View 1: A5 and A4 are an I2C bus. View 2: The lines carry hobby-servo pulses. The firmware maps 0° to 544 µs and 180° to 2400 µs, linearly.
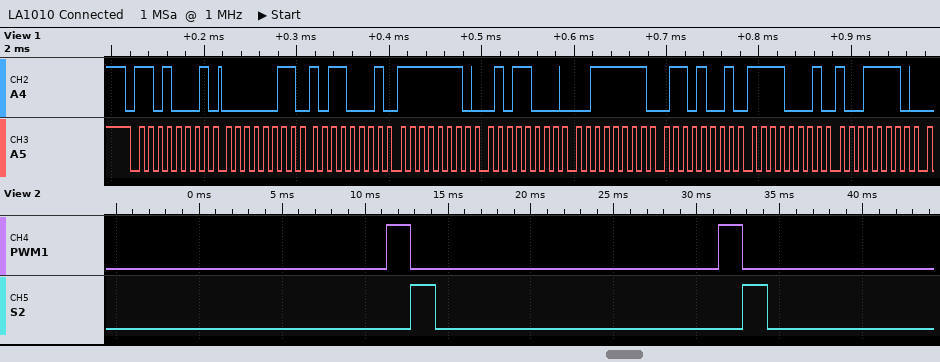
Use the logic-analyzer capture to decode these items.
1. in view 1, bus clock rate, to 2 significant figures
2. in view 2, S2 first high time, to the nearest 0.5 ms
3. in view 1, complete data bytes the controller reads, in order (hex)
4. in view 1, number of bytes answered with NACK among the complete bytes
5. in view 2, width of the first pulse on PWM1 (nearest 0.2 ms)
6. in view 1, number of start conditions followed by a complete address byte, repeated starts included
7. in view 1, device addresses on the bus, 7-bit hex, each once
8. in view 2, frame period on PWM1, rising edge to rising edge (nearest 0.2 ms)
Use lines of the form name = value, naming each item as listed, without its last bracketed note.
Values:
in view 1, bus clock rate, to 2 significant figures = 100 kHz
in view 2, S2 first high time, to the nearest 0.5 ms = 1.5 ms
in view 1, complete data bytes the controller reads, in order = 03 B1 FE 58 3F 69 F1 9E
in view 1, number of bytes answered with NACK among the complete bytes = 0
in view 2, width of the first pulse on PWM1 = 1.4 ms
in view 1, number of start conditions followed by a complete address byte, repeated starts included = 1
in view 1, device addresses on the bus, 7-bit hex, each once = 0x68
in view 2, frame period on PWM1, rising edge to rising edge = 20.0 ms
